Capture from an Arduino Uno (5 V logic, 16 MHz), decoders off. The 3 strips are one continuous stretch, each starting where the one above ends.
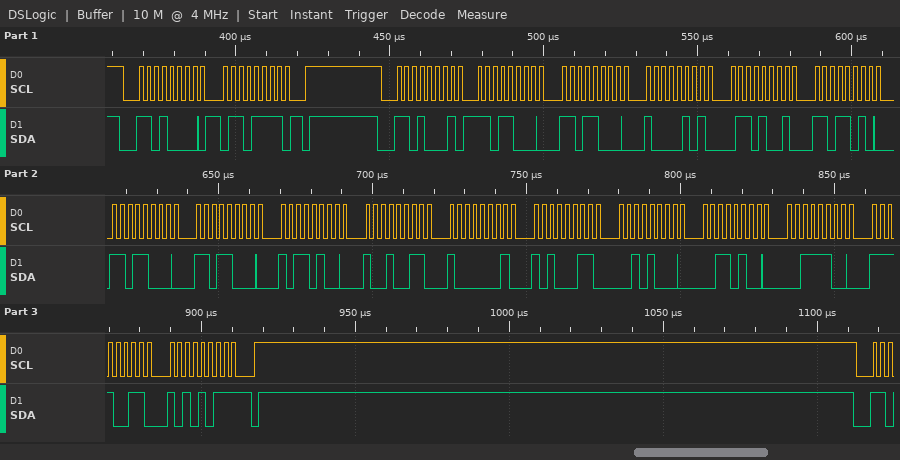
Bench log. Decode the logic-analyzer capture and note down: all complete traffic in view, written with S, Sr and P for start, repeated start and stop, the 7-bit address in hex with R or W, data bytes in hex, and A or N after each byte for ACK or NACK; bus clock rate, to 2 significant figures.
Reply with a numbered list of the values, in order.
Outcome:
1. S 68W A 6F A P S 68R A D8 A D8 A 85 A 69 A DA A D8 A D8 A B4 A 93 A 81 A A3 A 28 A 34 A 3C A F3 A AB N P
2. 400 kHz
